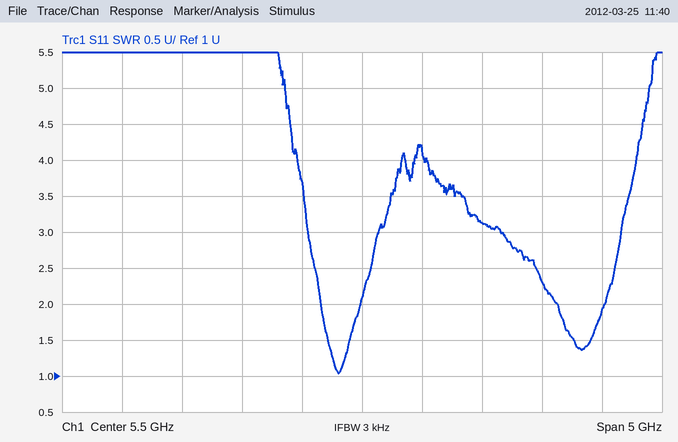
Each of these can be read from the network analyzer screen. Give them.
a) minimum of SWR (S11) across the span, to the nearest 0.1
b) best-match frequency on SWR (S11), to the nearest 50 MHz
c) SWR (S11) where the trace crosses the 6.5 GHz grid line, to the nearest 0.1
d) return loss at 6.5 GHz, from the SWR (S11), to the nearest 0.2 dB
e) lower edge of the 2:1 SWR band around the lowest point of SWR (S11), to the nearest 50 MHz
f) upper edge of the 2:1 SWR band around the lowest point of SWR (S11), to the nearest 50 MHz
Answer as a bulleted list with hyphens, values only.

- 1.0
- 5.30 GHz
- 3.1
- 5.8 dB
- 5.15 GHz
- 5.50 GHz
